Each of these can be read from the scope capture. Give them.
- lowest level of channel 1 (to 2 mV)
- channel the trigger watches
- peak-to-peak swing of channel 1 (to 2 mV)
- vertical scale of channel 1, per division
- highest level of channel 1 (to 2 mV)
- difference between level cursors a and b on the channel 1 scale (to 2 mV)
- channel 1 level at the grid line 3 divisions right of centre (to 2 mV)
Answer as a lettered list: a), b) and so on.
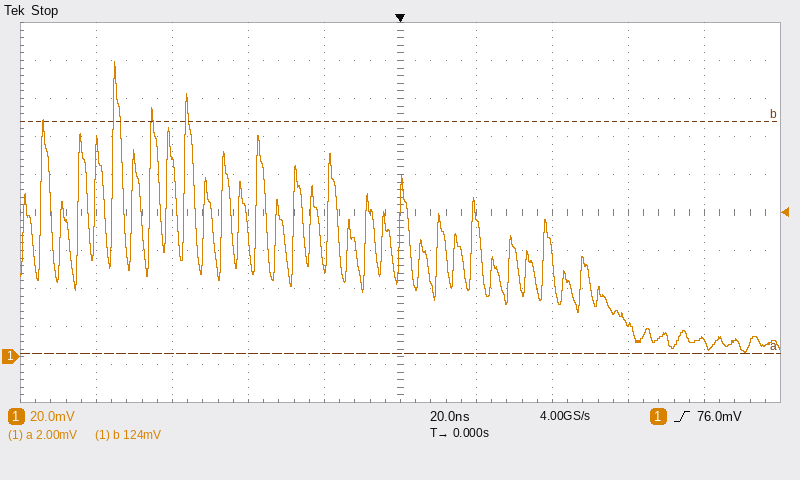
a) 2 mV
b) channel 1
c) 154 mV
d) 20 mV
e) 156 mV
f) 122 mV
g) 18 mV
